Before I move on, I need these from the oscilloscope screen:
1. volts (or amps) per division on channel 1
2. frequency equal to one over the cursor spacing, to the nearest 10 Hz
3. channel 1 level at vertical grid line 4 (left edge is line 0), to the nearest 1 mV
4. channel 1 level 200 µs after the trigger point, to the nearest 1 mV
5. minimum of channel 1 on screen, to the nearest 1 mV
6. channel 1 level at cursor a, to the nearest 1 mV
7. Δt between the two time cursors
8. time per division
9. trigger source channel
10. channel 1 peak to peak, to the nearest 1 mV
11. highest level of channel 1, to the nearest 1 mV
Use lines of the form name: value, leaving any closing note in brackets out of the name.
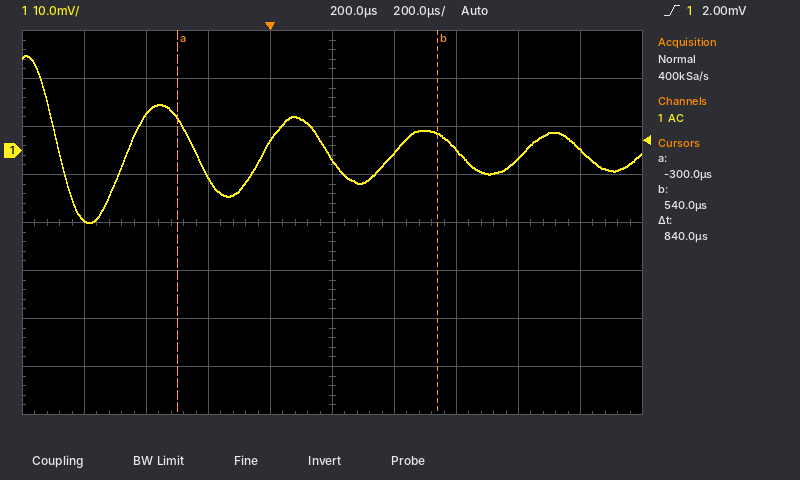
volts (or amps) per division on channel 1: 10 mV
frequency equal to one over the cursor spacing, to the nearest 10 Hz: 1.19 kHz
channel 1 level at vertical grid line 4 (left edge is line 0), to the nearest 1 mV: 2 mV
channel 1 level 200 µs after the trigger point, to the nearest 1 mV: -2 mV
minimum of channel 1 on screen, to the nearest 1 mV: -15 mV
channel 1 level at cursor a, to the nearest 1 mV: 7 mV
Δt between the two time cursors: 840 µs
time per division: 200 µs
trigger source channel: channel 1
channel 1 peak to peak, to the nearest 1 mV: 35 mV
highest level of channel 1, to the nearest 1 mV: 20 mV
